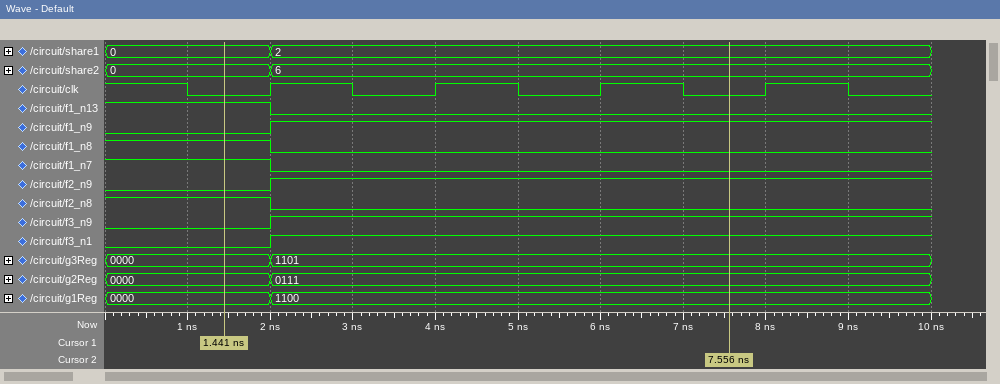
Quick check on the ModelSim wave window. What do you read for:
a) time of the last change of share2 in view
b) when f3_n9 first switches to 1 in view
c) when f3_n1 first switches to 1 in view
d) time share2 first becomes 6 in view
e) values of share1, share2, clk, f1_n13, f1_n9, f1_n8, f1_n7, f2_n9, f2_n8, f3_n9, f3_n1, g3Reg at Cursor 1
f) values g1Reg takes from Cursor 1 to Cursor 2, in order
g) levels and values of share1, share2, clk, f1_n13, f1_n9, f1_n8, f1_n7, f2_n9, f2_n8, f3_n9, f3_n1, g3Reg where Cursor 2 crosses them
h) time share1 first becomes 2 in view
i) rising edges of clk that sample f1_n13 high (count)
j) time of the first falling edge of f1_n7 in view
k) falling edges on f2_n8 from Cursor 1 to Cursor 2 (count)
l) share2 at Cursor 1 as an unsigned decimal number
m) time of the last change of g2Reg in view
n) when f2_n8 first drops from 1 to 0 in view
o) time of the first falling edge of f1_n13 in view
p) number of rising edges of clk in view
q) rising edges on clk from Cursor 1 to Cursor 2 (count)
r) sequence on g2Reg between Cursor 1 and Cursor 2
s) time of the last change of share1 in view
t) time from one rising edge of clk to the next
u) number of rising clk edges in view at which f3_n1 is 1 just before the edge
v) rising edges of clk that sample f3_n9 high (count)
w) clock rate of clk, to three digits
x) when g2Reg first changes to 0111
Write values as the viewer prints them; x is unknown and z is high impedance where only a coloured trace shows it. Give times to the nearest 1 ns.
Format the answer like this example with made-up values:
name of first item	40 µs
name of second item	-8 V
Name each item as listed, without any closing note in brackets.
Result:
time of the last change of share2 in view	2 ns
when f3_n9 first switches to 1 in view	2 ns
when f3_n1 first switches to 1 in view	2 ns
time share2 first becomes 6 in view	2 ns
values of share1, share2, clk, f1_n13, f1_n9, f1_n8, f1_n7, f2_n9, f2_n8, f3_n9, f3_n1, g3Reg at Cursor 1	share1=0, share2=0, clk=0, f1_n13=1, f1_n9=0, f1_n8=1, f1_n7=1, f2_n9=0, f2_n8=1, f3_n9=0, f3_n1=0, g3Reg=0000
values g1Reg takes from Cursor 1 to Cursor 2, in order	0000, 1100
levels and values of share1, share2, clk, f1_n13, f1_n9, f1_n8, f1_n7, f2_n9, f2_n8, f3_n9, f3_n1, g3Reg where Cursor 2 crosses them	share1=2, share2=6, clk=0, f1_n13=0, f1_n9=1, f1_n8=0, f1_n7=0, f2_n9=1, f2_n8=0, f3_n9=1, f3_n1=1, g3Reg=1101
time share1 first becomes 2 in view	2 ns
rising edges of clk that sample f1_n13 high	1
time of the first falling edge of f1_n7 in view	2 ns
falling edges on f2_n8 from Cursor 1 to Cursor 2	1
share2 at Cursor 1 as an unsigned decimal number	0
time of the last change of g2Reg in view	2 ns
when f2_n8 first drops from 1 to 0 in view	2 ns
time of the first falling edge of f1_n13 in view	2 ns
number of rising edges of clk in view	4
rising edges on clk from Cursor 1 to Cursor 2	3
sequence on g2Reg between Cursor 1 and Cursor 2	0000, 0111
time of the last change of share1 in view	2 ns
time from one rising edge of clk to the next	2 ns
number of rising clk edges in view at which f3_n1 is 1 just before the edge	3
rising edges of clk that sample f3_n9 high	3
clock rate of clk, to three digits	500 MHz
when g2Reg first changes to 0111	2 ns
